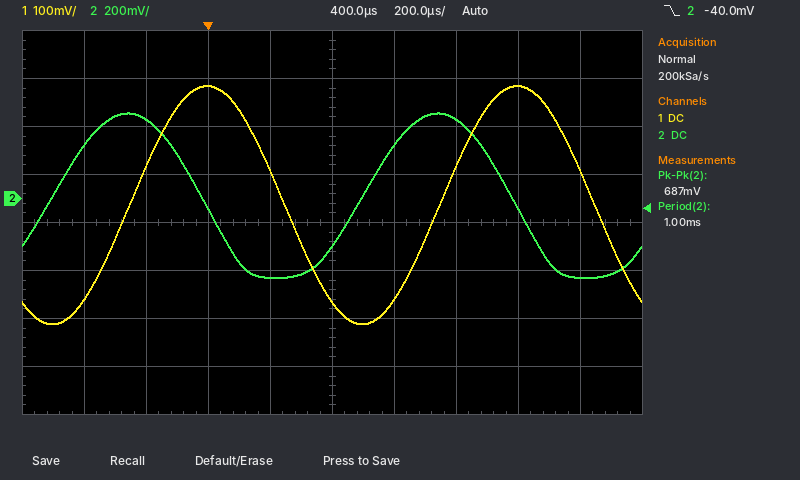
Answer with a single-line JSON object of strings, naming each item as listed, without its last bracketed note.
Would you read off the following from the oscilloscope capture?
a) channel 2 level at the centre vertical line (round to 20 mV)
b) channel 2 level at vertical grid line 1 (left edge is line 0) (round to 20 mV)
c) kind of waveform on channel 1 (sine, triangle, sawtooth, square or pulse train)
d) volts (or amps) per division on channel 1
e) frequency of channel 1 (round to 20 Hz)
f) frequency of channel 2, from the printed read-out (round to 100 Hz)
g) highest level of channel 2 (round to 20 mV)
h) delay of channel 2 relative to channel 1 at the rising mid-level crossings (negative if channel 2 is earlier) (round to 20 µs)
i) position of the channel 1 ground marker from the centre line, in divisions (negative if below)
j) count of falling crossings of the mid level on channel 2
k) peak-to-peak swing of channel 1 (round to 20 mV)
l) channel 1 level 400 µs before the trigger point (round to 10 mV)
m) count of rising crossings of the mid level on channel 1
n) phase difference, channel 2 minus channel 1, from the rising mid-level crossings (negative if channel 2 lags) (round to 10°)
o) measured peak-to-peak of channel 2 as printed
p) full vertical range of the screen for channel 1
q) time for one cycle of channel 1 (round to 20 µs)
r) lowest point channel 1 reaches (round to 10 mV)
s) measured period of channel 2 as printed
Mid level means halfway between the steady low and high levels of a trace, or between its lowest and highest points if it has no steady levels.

{"channel 2 level at the centre vertical line": "-200 mV", "channel 2 level at vertical grid line 1 (left edge is line 0)": "220 mV", "kind of waveform on channel 1": "sine", "volts (or amps) per division on channel 1": "100 mV", "frequency of channel 1": "1.00 kHz", "frequency of channel 2, from the printed read-out": "1.0 kHz", "highest level of channel 2": "360 mV", "delay of channel 2 relative to channel 1 at the rising mid-level crossings (negative if channel 2 is earlier)": "-240 µs", "position of the channel 1 ground marker from the centre line, in divisions": "+0.5 div", "count of falling crossings of the mid level on channel 2": "2", "peak-to-peak swing of channel 1": "500 mV", "channel 1 level 400 µs before the trigger point": "-210 mV", "count of rising crossings of the mid level on channel 1": "2", "phase difference, channel 2 minus channel 1, from the rising mid-level crossings (negative if channel 2 lags)": "+90°", "measured peak-to-peak of channel 2 as printed": "687 mV", "full vertical range of the screen for channel 1": "800 mV", "time for one cycle of channel 1": "1.00 ms", "lowest point channel 1 reaches": "-260 mV", "measured period of channel 2 as printed": "1.00 ms"}
